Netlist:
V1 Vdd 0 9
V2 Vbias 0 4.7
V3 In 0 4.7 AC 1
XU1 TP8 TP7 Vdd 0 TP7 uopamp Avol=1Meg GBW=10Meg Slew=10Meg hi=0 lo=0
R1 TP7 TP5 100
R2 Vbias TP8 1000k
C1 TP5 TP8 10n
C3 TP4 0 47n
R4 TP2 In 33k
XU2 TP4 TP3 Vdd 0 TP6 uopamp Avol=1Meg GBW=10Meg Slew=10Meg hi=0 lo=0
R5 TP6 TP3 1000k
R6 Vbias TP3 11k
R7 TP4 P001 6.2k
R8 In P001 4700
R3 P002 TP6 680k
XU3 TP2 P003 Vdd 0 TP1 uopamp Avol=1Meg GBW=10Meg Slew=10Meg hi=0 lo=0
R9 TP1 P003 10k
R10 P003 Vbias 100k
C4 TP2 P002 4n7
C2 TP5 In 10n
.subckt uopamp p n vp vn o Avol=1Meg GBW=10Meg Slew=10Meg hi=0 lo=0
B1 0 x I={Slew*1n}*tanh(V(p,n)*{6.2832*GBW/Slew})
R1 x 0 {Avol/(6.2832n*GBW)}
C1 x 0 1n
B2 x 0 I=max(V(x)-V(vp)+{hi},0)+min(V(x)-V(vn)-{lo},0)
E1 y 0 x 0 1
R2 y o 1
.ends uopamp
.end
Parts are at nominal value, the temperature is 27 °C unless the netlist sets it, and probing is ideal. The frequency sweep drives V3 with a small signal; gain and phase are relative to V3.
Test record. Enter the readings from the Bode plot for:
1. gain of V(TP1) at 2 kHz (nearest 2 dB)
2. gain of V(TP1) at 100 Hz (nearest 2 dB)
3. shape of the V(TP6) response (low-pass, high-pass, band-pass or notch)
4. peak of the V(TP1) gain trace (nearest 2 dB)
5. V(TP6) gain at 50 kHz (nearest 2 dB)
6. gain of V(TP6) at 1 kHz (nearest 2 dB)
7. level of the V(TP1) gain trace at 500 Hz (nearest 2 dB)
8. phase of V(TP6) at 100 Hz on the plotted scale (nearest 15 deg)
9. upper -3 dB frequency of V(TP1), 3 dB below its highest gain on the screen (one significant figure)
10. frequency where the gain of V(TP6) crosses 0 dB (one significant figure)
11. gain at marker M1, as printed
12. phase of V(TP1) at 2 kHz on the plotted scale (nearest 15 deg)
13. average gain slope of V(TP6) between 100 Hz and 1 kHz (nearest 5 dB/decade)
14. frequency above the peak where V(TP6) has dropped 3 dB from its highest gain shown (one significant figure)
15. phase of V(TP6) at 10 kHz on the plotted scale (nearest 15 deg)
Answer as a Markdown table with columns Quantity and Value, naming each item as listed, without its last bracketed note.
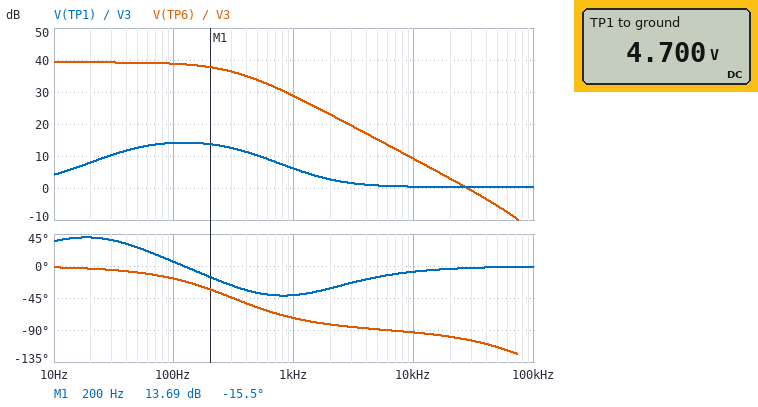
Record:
| Quantity | Value |
|---|---|
| gain of V(TP1) at 2 kHz | 2 dB |
| gain of V(TP1) at 100 Hz | 14 dB |
| shape of the V(TP6) response | low-pass |
| peak of the V(TP1) gain trace | 14 dB |
| V(TP6) gain at 50 kHz | -6 dB |
| gain of V(TP6) at 1 kHz | 28 dB |
| level of the V(TP1) gain trace at 500 Hz | 10 dB |
| phase of V(TP6) at 100 Hz on the plotted scale | -15 deg |
| upper -3 dB frequency of V(TP1), 3 dB below its highest gain on the screen | 400 Hz |
| frequency where the gain of V(TP6) crosses 0 dB | 30 kHz |
| gain at marker M1, as printed | 13.69 dB |
| phase of V(TP1) at 2 kHz on the plotted scale | -30 deg |
| average gain slope of V(TP6) between 100 Hz and 1 kHz | -10 dB/decade |
| frequency above the peak where V(TP6) has dropped 3 dB from its highest gain shown | 300 Hz |
| phase of V(TP6) at 10 kHz on the plotted scale | -90 deg |
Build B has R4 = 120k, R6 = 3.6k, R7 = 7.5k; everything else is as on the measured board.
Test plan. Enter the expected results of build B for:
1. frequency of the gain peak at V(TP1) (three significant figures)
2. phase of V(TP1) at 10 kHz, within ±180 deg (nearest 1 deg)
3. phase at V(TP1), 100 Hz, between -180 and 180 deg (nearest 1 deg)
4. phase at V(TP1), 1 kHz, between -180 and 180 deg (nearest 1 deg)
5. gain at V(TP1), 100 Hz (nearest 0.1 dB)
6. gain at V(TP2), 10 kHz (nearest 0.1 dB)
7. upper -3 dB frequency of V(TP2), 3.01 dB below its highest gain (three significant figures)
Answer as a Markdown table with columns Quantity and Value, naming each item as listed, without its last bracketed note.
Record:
| Quantity | Value |
|---|---|
| frequency of the gain peak at V(TP1) | 108 Hz |
| phase of V(TP1) at 10 kHz, within ±180 deg | -62 deg |
| phase at V(TP1), 100 Hz, between -180 and 180 deg | 3 deg |
| phase at V(TP1), 1 kHz, between -180 and 180 deg | -70 deg |
| gain at V(TP1), 100 Hz | 32.2 dB |
| gain at V(TP2), 10 kHz | 1.8 dB |
| upper -3 dB frequency of V(TP2), 3.01 dB below its highest gain | 353 Hz |
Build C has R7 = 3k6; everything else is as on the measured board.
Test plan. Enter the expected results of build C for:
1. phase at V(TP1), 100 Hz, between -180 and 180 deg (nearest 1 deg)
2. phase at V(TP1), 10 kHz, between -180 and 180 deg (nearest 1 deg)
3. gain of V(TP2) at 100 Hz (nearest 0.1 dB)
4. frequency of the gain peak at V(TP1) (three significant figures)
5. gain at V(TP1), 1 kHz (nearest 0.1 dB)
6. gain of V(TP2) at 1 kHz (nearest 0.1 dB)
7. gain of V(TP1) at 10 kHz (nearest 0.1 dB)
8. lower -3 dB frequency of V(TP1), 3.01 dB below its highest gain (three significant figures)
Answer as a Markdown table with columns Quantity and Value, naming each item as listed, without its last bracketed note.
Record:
| Quantity | Value |
|---|---|
| phase at V(TP1), 100 Hz, between -180 and 180 deg | 9 deg |
| phase at V(TP1), 10 kHz, between -180 and 180 deg | -10 deg |
| gain of V(TP2) at 100 Hz | 13.4 dB |
| frequency of the gain peak at V(TP1) | 139 Hz |
| gain at V(TP1), 1 kHz | 7.6 dB |
| gain of V(TP2) at 1 kHz | 6.8 dB |
| gain of V(TP1) at 10 kHz | 0.5 dB |
| lower -3 dB frequency of V(TP1), 3.01 dB below its highest gain | 37.6 Hz |
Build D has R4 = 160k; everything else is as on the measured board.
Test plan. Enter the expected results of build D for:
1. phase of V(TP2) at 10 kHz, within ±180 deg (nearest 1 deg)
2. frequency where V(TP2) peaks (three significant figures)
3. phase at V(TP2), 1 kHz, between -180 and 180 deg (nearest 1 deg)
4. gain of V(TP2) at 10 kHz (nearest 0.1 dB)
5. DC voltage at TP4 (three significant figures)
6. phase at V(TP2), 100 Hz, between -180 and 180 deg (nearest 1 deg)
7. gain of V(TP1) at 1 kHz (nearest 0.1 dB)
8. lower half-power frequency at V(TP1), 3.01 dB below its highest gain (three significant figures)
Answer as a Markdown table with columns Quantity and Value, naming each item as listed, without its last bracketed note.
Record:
| Quantity | Value |
|---|---|
| phase of V(TP2) at 10 kHz, within ±180 deg | -35 deg |
| frequency where V(TP2) peaks | 112 Hz |
| phase at V(TP2), 1 kHz, between -180 and 180 deg | -63 deg |
| gain of V(TP2) at 10 kHz | -0.5 dB |
| DC voltage at TP4 | 4.70 V |
| phase at V(TP2), 100 Hz, between -180 and 180 deg | 4 deg |
| gain of V(TP1) at 1 kHz | 15.7 dB |
| lower half-power frequency at V(TP1), 3.01 dB below its highest gain | 32.5 Hz |
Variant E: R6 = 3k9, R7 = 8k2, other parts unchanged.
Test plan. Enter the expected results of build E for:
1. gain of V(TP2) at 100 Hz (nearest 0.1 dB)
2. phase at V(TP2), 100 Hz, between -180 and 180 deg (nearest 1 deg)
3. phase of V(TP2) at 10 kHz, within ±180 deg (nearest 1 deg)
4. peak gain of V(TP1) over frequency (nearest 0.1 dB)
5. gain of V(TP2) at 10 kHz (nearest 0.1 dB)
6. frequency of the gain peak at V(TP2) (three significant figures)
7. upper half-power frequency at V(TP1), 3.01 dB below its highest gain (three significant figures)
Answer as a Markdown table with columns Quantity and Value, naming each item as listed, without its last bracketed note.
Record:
| Quantity | Value |
|---|---|
| gain of V(TP2) at 100 Hz | 20.8 dB |
| phase at V(TP2), 100 Hz, between -180 and 180 deg | 4 deg |
| phase of V(TP2) at 10 kHz, within ±180 deg | -18 deg |
| peak gain of V(TP1) over frequency | 21.7 dB |
| gain of V(TP2) at 10 kHz | -0.6 dB |
| frequency of the gain peak at V(TP2) | 112 Hz |
| upper half-power frequency at V(TP1), 3.01 dB below its highest gain | 348 Hz |
